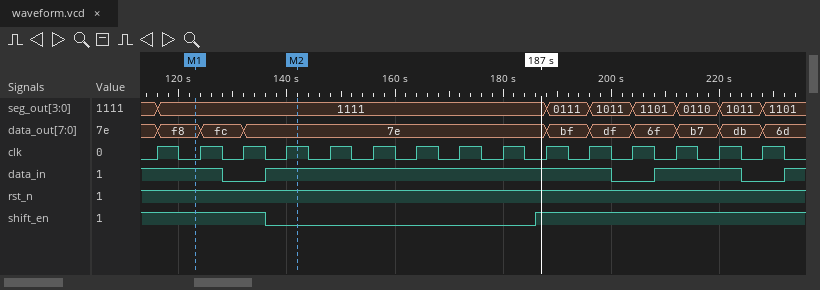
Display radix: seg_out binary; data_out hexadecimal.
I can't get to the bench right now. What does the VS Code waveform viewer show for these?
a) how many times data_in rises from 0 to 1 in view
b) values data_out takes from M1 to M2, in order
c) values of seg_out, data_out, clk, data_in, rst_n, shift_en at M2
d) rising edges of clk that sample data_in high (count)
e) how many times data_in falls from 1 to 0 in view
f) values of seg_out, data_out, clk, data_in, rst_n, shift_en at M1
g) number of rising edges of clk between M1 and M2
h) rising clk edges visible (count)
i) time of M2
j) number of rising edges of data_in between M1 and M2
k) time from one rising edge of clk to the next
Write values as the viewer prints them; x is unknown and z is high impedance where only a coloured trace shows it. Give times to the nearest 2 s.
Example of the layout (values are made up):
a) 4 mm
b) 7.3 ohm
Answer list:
a) 3
b) f8, fc, 7e
c) seg_out=1111, data_out=7e, clk=1, data_in=1, rst_n=1, shift_en=0
d) 12
e) 3
f) seg_out=1111, data_out=f8, clk=0, data_in=1, rst_n=1, shift_en=1
g) 3
h) 15
i) 142 s
j) 1
k) 8 s
